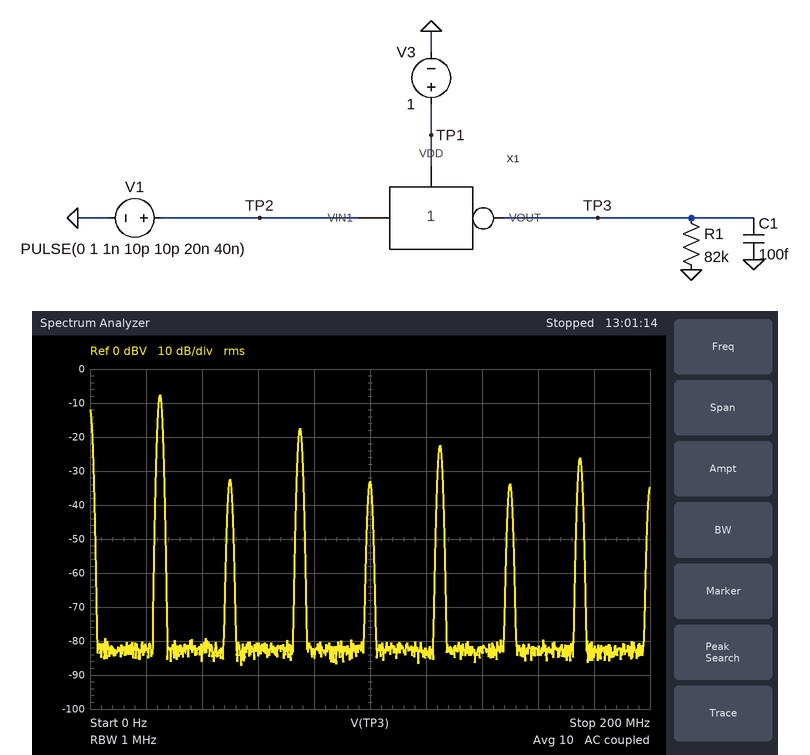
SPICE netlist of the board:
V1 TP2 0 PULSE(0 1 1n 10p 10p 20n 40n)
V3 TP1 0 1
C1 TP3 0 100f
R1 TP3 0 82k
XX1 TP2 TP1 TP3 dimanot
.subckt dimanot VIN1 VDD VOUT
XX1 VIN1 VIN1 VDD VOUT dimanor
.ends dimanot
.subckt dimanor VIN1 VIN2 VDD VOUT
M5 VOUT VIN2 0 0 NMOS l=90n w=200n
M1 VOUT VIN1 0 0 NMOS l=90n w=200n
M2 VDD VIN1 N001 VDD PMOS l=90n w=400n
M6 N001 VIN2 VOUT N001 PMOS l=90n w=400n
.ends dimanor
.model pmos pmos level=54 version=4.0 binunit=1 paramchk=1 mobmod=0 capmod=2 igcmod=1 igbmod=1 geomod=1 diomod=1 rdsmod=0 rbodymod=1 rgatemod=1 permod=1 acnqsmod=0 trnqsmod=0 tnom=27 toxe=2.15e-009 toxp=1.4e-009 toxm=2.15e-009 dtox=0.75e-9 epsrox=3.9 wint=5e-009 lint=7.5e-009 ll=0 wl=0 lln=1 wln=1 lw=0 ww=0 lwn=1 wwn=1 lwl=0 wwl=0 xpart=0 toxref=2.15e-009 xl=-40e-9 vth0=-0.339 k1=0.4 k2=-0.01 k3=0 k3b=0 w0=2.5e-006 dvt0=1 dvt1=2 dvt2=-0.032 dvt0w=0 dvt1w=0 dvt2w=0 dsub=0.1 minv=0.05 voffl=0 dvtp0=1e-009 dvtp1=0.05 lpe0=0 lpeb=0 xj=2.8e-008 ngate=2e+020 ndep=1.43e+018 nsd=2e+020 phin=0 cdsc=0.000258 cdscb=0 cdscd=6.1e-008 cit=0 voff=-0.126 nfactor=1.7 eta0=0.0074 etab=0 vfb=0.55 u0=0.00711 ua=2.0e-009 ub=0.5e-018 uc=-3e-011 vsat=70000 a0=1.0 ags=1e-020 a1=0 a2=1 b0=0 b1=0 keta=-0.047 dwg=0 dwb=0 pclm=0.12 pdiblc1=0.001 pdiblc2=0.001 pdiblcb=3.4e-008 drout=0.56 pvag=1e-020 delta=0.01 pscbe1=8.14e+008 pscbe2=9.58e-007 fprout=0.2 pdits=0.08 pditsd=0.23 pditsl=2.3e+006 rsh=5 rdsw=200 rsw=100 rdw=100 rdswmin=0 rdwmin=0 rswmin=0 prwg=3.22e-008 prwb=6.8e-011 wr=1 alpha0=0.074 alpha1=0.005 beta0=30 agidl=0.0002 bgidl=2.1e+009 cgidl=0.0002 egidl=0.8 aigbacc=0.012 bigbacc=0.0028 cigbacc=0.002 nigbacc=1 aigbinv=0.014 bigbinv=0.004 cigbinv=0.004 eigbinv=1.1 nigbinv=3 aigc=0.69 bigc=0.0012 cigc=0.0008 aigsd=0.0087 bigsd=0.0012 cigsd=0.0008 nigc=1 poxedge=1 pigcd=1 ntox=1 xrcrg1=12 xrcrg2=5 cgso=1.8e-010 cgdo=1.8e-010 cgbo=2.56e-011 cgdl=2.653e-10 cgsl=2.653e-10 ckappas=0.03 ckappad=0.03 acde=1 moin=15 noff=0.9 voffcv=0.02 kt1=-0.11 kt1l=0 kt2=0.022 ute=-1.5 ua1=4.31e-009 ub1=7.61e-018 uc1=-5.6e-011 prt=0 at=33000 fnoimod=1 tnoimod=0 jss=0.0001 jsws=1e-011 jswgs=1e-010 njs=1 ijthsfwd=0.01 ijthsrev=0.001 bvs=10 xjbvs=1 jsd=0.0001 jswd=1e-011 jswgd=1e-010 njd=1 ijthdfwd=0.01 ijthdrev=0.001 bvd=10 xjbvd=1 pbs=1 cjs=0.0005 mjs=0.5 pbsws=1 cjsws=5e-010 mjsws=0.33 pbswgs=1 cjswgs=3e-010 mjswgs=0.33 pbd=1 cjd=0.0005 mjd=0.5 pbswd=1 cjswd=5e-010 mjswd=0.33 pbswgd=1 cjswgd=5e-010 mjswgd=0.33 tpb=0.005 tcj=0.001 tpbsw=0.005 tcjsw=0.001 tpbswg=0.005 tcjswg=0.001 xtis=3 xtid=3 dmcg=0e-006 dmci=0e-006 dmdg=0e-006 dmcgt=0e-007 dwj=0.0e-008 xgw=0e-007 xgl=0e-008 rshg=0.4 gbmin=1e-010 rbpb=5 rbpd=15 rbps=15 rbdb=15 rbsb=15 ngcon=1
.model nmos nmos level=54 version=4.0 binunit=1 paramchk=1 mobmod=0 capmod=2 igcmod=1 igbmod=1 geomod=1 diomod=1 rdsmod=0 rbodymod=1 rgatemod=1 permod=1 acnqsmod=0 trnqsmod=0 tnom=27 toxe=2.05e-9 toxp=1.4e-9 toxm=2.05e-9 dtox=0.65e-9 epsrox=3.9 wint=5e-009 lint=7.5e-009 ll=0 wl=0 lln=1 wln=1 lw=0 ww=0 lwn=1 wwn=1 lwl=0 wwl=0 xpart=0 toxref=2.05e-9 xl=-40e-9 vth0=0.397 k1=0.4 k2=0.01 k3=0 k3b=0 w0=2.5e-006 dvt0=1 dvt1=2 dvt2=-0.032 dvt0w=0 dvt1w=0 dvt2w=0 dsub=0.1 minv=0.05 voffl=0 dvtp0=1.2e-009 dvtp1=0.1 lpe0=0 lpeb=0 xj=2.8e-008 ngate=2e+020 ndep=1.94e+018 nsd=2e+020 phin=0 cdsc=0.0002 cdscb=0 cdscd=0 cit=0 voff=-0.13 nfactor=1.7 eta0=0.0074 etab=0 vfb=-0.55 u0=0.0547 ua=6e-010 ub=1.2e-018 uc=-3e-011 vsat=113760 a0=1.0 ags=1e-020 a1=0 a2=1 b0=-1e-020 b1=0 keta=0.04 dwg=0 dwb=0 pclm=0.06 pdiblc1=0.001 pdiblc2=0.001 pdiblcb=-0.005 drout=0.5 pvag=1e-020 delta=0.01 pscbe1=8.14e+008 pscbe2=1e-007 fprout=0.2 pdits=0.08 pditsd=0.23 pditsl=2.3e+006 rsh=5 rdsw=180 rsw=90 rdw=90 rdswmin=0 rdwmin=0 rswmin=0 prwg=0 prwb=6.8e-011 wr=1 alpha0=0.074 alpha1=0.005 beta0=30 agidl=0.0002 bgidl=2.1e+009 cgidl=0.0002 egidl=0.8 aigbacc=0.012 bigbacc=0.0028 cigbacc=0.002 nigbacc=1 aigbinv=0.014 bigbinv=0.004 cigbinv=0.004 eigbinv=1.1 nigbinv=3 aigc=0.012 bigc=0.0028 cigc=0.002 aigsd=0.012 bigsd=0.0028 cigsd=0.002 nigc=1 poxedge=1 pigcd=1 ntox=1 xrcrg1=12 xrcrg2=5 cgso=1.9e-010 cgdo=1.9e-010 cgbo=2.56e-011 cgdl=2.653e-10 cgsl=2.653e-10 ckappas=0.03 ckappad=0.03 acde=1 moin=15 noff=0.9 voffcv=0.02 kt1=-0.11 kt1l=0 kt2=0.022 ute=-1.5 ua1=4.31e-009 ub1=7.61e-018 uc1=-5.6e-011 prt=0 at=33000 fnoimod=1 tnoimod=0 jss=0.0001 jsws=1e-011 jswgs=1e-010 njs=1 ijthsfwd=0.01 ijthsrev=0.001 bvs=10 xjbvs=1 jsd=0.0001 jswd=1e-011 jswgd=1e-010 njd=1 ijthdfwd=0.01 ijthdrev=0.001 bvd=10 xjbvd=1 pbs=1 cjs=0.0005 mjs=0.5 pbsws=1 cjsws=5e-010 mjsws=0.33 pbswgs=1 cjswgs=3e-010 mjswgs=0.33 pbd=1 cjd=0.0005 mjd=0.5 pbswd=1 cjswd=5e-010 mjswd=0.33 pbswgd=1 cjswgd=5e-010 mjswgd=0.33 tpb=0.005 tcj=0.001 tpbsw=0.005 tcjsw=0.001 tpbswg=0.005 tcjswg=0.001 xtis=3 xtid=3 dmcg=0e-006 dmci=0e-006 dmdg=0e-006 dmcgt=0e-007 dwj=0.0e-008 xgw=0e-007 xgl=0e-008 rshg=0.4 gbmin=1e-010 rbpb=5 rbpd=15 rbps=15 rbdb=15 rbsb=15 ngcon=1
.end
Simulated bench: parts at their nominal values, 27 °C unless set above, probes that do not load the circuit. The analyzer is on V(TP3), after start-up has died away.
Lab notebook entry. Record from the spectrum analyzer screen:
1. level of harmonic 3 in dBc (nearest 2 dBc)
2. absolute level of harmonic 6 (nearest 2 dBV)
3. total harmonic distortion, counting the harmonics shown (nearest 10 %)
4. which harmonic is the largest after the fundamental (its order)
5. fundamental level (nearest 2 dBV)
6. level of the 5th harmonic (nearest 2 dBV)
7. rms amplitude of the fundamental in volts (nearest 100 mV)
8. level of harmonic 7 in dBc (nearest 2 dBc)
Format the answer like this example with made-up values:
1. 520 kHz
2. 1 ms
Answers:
1. -10 dBc
2. -34 dBV
3. 40 %
4. 3
5. -8 dBV
6. -22 dBV
7. 400 mV
8. -18 dBc
